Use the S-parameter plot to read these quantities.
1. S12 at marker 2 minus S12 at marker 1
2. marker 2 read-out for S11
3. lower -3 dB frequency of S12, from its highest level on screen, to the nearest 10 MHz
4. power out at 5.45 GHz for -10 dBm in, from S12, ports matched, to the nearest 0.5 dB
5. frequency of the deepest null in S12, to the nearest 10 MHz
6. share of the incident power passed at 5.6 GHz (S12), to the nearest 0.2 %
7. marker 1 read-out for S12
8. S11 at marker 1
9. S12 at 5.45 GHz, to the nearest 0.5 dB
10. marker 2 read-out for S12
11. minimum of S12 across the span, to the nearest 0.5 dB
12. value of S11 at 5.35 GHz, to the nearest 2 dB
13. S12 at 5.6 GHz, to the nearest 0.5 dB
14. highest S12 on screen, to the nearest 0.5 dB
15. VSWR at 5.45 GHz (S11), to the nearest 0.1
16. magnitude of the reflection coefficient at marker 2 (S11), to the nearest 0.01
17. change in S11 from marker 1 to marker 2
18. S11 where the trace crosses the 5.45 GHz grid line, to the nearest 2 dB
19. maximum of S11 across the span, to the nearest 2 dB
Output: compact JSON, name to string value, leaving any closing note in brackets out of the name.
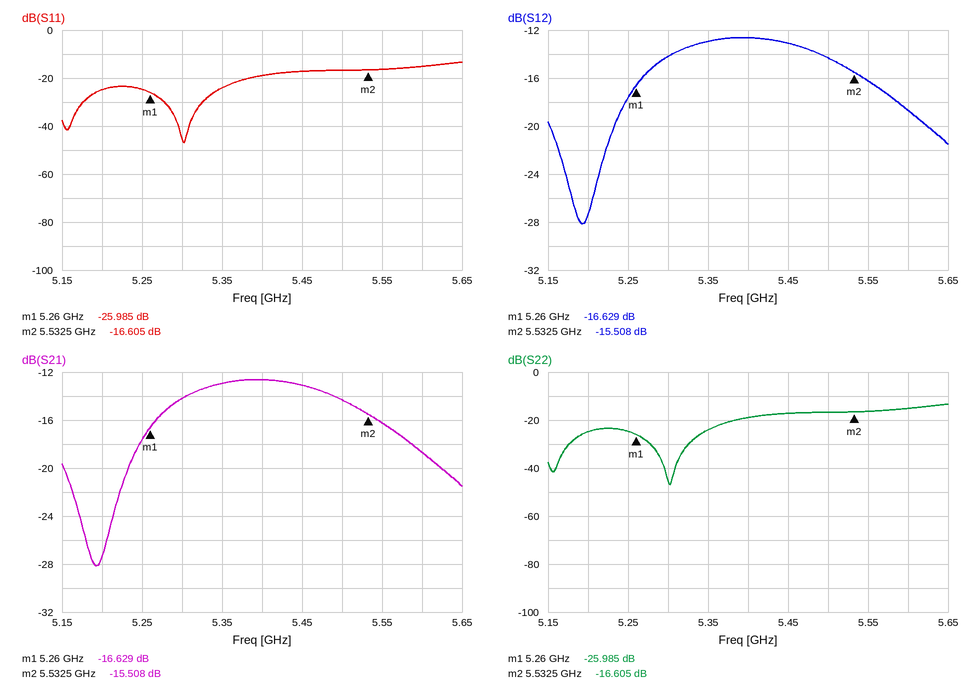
{"S12 at marker 2 minus S12 at marker 1": "1.121 dB", "marker 2 read-out for S11": "-16.605 dB", "lower -3 dB frequency of S12, from its highest level on screen, to the nearest 10 MHz": "5.27 GHz", "power out at 5.45 GHz for -10 dBm in, from S12, ports matched, to the nearest 0.5 dB": "-23.0 dBm", "frequency of the deepest null in S12, to the nearest 10 MHz": "5.19 GHz", "share of the incident power passed at 5.6 GHz (S12), to the nearest 0.2 %": "1.4 %", "marker 1 read-out for S12": "-16.629 dB", "S11 at marker 1": "-25.985 dB", "S12 at 5.45 GHz, to the nearest 0.5 dB": "-13.0 dB", "marker 2 read-out for S12": "-15.508 dB", "minimum of S12 across the span, to the nearest 0.5 dB": "-28.0 dB", "value of S11 at 5.35 GHz, to the nearest 2 dB": "-24 dB", "S12 at 5.6 GHz, to the nearest 0.5 dB": "-18.5 dB", "highest S12 on screen, to the nearest 0.5 dB": "-12.5 dB", "VSWR at 5.45 GHz (S11), to the nearest 0.1": "1.3", "magnitude of the reflection coefficient at marker 2 (S11), to the nearest 0.01": "0.15", "change in S11 from marker 1 to marker 2": "9.380 dB", "S11 where the trace crosses the 5.45 GHz grid line, to the nearest 2 dB": "-18 dB", "maximum of S11 across the span, to the nearest 2 dB": "-14 dB"}
